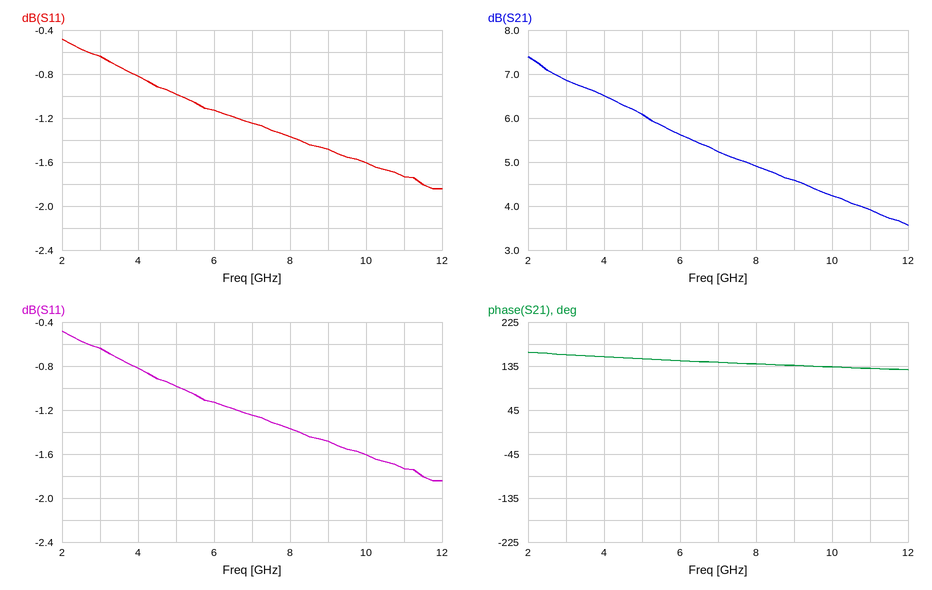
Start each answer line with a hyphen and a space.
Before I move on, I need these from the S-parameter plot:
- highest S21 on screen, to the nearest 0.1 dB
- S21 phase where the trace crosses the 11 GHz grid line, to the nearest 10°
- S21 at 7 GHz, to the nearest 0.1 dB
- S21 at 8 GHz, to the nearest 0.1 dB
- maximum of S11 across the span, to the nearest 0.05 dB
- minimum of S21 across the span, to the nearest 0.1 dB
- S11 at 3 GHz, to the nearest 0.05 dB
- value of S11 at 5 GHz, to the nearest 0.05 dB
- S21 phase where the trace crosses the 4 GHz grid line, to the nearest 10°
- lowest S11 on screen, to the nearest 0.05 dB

- 7.4 dB
- 130°
- 5.2 dB
- 4.9 dB
- -0.50 dB
- 3.6 dB
- -0.65 dB
- -1.00 dB
- 150°
- -1.85 dB
